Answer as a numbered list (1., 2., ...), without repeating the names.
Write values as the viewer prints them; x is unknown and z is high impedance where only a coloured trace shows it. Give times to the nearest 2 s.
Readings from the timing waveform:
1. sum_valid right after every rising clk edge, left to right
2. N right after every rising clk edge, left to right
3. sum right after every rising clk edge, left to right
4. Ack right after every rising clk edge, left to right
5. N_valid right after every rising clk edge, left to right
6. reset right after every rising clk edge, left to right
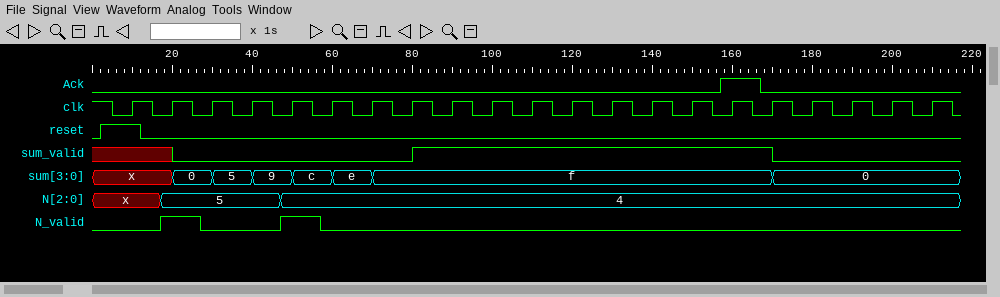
1. x 0 0 0 0 0 0 1 1 1 1 1 1 1 1 1 0 0 0 0 0
2. x, 5, 5, 5, 4, 4, 4, 4, 4, 4, 4, 4, 4, 4, 4, 4, 4, 4, 4, 4, 4
3. x, 0, 5, 9, c, e, f, f, f, f, f, f, f, f, f, f, 0, 0, 0, 0, 0
4. 0 0 0 0 0 0 0 0 0 0 0 0 0 0 0 1 0 0 0 0 0
5. 0 1 0 0 1 0 0 0 0 0 0 0 0 0 0 0 0 0 0 0 0
6. 1 0 0 0 0 0 0 0 0 0 0 0 0 0 0 0 0 0 0 0 0
